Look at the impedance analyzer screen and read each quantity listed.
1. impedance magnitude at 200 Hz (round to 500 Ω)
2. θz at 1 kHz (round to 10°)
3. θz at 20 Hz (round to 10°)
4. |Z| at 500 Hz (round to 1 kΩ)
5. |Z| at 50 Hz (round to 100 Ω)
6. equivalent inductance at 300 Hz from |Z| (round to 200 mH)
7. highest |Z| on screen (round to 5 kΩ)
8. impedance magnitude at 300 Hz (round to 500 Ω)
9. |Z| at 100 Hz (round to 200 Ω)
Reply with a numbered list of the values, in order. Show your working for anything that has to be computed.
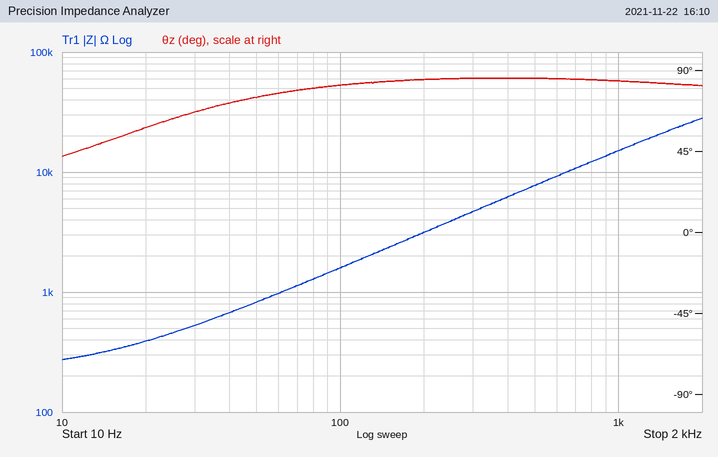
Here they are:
1. 3.0 kΩ
2. 80°
3. 60°
4. 8 kΩ
5. 800 Ω
6. L = 4.5 kΩ/(2π × 300 Hz) ≈ 2.4 H
7. 30 kΩ
8. 4.5 kΩ
9. 1.6 kΩ
